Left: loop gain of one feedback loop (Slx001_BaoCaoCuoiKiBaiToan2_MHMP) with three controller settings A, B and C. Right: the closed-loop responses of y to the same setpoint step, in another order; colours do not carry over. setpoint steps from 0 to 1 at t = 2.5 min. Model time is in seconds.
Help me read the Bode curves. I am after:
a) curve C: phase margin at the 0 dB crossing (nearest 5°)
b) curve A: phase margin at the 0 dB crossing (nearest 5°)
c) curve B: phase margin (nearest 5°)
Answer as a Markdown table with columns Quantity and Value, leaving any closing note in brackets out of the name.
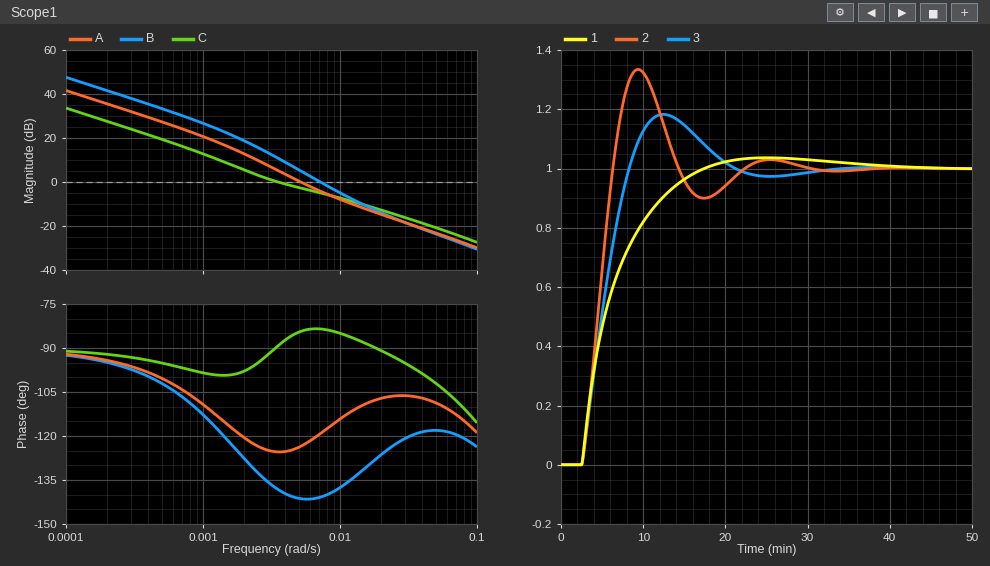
| Quantity | Value |
|---|---|
| curve C: phase margin at the 0 dB crossing | 90° |
| curve A: phase margin at the 0 dB crossing | 55° |
| curve B: phase margin | 40° |
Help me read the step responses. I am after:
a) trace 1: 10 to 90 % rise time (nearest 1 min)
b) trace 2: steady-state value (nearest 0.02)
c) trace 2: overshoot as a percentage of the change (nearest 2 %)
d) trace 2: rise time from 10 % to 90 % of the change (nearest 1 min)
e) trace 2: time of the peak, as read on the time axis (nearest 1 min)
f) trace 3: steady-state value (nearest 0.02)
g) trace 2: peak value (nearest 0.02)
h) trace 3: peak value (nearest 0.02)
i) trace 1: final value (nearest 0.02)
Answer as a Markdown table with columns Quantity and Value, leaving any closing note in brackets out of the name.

| Quantity | Value |
|---|---|
| trace 1: 10 to 90 % rise time | 9 min |
| trace 2: steady-state value | 1.00 |
| trace 2: overshoot as a percentage of the change | 34 % |
| trace 2: rise time from 10 % to 90 % of the change | 3 min |
| trace 2: time of the peak, as read on the time axis | 9 min |
| trace 3: steady-state value | 1.00 |
| trace 2: peak value | 1.34 |
| trace 3: peak value | 1.18 |
| trace 1: final value | 1.00 |
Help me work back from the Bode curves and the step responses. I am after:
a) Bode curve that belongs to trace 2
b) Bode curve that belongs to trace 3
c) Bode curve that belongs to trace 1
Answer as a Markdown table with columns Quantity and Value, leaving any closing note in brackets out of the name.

| Quantity | Value |
|---|---|
| Bode curve that belongs to trace 2 | B |
| Bode curve that belongs to trace 3 | A |
| Bode curve that belongs to trace 1 | C |
